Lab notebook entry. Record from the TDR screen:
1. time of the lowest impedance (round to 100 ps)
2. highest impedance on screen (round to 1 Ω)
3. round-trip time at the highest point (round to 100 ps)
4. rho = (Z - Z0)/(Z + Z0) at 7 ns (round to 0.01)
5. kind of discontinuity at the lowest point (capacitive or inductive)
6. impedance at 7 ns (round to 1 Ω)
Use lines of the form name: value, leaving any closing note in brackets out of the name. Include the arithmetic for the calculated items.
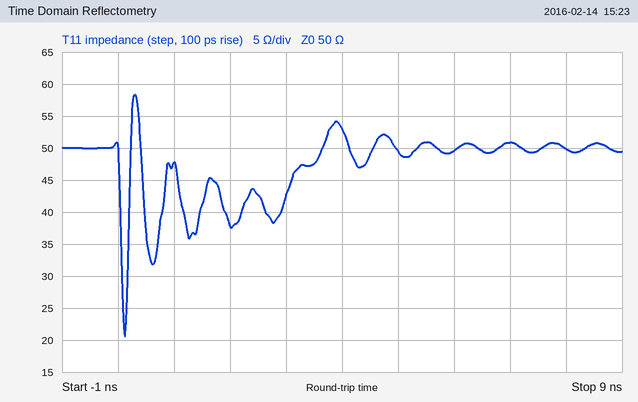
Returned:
time of the lowest impedance: 100 ps
highest impedance on screen: 58 Ω
round-trip time at the highest point: 300 ps
rho = (Z - Z0)/(Z + Z0) at 7 ns: (51 − 50)/(51 + 50) ≈ +0.01
kind of discontinuity at the lowest point: capacitive
impedance at 7 ns: 51 Ω
